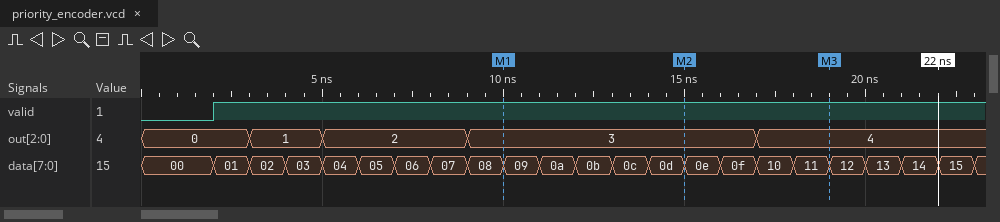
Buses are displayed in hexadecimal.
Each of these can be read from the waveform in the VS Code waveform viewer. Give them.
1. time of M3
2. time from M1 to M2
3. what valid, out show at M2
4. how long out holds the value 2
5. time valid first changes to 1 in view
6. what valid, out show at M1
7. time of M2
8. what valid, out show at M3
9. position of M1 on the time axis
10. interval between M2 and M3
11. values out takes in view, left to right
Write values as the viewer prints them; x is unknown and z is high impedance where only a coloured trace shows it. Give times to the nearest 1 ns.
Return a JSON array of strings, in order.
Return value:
["19 ns", "5 ns", "valid=1, out=3", "4 ns", "2 ns", "valid=1, out=3", "15 ns", "valid=1, out=4", "10 ns", "4 ns", "0, 1, 2, 3, 4"]
